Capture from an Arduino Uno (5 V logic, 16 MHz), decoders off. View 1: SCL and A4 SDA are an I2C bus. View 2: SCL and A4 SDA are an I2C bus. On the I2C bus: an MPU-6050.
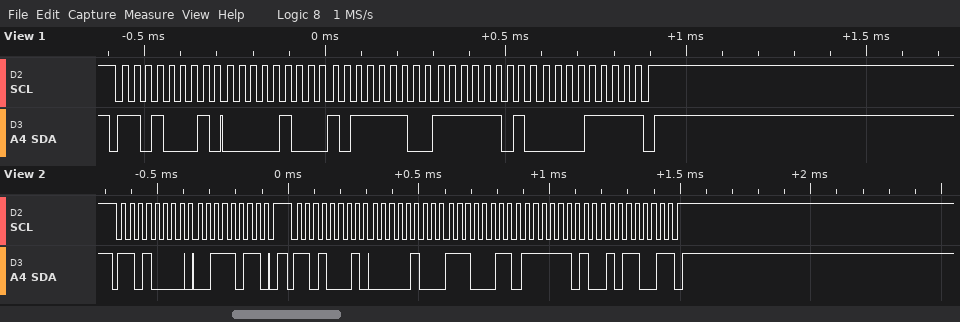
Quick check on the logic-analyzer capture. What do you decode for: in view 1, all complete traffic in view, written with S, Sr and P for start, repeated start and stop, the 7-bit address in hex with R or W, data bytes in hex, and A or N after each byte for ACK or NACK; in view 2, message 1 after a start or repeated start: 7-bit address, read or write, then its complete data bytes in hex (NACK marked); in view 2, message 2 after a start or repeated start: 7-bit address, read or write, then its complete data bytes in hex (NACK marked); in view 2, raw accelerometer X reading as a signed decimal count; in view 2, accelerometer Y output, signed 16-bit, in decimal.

S 68R A 04 A BE A FD A 0F N P
0x68 write: 3B
0x68 read: 04 E3 FD 59 NACK
1251
-679
